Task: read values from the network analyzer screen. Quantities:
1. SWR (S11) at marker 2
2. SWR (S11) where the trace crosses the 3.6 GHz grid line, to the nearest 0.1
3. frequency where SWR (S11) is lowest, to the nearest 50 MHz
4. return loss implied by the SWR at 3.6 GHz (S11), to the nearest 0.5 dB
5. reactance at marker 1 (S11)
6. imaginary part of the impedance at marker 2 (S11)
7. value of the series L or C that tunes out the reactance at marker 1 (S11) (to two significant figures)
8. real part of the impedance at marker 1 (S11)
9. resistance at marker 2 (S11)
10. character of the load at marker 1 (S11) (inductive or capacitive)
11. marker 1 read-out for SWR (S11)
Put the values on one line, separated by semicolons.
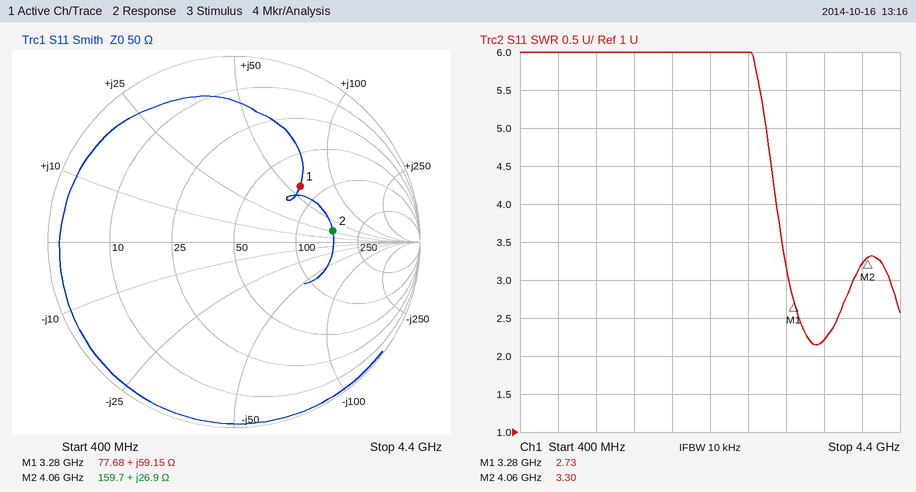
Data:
3.30; 2.2; 3.50 GHz; 8.5 dB; +59.15 Ω; +26.9 Ω; 820 fF; 77.68 Ω; 159.7 Ω; inductive; 2.73
